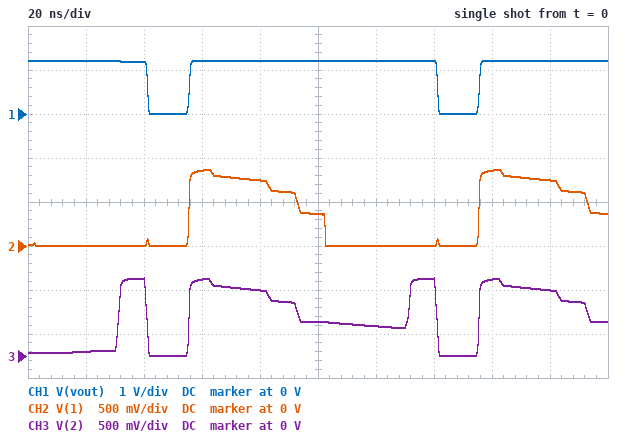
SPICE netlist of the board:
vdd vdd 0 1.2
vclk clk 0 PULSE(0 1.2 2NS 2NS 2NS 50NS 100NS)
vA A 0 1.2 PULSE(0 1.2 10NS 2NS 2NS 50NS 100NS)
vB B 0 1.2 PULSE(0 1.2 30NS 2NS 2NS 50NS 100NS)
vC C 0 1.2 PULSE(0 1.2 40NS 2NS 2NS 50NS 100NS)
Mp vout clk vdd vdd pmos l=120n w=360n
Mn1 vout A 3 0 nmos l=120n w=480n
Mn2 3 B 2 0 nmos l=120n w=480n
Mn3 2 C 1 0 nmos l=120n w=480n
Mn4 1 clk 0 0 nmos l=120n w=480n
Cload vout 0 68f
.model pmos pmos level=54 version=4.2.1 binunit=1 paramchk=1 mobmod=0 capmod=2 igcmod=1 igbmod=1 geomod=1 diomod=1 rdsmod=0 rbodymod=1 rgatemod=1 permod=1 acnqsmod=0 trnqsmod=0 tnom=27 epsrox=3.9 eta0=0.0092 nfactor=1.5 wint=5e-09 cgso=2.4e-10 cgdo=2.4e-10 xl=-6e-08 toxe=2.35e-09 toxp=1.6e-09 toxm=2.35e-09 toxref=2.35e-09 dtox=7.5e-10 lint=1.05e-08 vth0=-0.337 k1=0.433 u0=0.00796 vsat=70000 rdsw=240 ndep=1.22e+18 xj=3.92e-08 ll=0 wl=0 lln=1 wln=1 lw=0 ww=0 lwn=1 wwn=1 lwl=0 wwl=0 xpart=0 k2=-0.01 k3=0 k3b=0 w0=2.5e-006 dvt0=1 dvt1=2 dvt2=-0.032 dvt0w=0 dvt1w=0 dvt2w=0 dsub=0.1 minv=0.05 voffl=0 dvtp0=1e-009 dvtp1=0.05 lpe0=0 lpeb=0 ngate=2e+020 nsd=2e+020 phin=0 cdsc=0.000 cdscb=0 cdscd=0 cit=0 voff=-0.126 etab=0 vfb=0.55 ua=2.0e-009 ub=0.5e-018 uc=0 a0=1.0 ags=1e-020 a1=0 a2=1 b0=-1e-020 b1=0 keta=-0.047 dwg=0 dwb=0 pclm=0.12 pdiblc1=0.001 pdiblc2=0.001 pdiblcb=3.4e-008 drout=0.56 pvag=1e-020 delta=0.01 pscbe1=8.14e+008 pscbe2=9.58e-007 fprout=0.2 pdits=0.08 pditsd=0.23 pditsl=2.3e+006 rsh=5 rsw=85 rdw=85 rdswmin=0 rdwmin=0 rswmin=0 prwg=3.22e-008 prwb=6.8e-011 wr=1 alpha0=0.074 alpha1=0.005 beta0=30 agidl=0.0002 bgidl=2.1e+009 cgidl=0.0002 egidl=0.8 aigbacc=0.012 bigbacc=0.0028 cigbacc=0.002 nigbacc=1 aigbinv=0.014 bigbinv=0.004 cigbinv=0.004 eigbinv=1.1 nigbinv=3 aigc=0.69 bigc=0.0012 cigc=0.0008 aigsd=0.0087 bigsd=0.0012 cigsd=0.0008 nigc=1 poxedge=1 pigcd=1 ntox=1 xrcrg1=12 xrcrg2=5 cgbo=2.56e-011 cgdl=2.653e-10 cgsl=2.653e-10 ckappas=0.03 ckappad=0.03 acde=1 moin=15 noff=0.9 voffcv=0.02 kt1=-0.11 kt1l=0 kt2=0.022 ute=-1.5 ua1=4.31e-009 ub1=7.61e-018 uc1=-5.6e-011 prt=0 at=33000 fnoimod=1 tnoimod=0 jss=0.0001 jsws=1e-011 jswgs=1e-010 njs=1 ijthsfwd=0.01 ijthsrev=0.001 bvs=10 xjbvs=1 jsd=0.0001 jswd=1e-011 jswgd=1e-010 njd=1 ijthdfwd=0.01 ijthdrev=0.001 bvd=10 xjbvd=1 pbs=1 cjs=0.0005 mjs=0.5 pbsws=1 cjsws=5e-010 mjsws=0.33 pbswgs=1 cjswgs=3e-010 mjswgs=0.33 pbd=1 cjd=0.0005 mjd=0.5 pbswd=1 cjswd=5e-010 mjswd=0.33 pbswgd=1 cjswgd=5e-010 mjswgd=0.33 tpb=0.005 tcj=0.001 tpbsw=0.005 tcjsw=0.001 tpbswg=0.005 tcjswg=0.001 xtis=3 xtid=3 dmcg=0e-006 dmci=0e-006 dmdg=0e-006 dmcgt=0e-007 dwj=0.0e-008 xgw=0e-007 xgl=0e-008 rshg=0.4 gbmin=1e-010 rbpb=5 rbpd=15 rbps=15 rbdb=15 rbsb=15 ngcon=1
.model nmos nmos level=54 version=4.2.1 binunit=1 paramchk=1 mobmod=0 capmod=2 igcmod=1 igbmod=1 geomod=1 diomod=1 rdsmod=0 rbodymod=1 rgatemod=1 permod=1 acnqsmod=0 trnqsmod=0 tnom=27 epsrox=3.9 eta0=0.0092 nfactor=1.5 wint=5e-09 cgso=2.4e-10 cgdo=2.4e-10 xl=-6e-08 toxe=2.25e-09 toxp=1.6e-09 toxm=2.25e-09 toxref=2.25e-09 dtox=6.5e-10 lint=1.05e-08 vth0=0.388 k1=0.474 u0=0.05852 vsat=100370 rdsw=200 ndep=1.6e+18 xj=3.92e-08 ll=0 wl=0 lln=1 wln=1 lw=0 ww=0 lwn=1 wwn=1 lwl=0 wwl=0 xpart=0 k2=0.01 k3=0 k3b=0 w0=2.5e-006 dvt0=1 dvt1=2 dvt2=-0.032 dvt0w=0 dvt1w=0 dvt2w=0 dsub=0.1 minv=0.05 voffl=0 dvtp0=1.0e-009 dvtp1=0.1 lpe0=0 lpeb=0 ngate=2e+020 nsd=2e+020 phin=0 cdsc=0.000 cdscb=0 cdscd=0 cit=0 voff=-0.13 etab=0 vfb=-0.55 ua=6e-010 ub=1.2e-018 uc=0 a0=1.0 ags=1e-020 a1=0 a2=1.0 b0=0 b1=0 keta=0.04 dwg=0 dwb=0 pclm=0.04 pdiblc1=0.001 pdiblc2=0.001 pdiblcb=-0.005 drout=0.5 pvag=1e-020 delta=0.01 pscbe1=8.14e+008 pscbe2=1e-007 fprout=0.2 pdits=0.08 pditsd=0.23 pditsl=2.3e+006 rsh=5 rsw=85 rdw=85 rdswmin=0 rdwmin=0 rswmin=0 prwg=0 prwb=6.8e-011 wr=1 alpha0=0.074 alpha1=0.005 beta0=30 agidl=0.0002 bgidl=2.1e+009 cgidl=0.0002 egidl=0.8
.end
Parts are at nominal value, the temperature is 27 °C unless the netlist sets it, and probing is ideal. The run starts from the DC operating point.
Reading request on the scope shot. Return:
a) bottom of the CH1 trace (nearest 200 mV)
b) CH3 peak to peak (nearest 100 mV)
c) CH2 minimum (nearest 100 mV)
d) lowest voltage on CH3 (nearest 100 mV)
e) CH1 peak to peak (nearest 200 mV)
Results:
0 V
900 mV
0 V
0 V
1.2 V
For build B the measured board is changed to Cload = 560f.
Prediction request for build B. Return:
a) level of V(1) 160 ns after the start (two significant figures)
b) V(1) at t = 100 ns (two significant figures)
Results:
830 mV
350 mV
